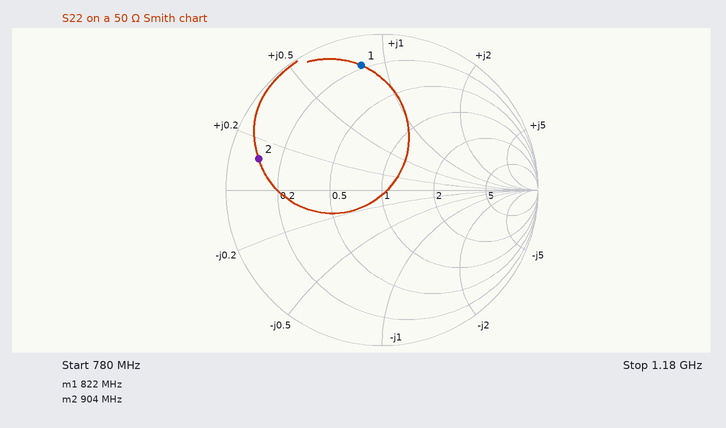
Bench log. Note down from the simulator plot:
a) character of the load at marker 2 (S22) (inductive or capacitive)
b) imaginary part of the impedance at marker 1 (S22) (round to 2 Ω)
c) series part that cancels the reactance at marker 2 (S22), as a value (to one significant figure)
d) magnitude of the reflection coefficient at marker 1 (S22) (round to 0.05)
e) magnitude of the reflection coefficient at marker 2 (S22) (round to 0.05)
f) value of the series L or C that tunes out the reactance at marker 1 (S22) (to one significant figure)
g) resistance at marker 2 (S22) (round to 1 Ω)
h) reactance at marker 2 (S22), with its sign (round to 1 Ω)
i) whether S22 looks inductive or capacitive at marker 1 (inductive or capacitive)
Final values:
inductive
+42 Ω
30 pF
0.80
0.80
5 pF
5 Ω
+6 Ω
inductive
